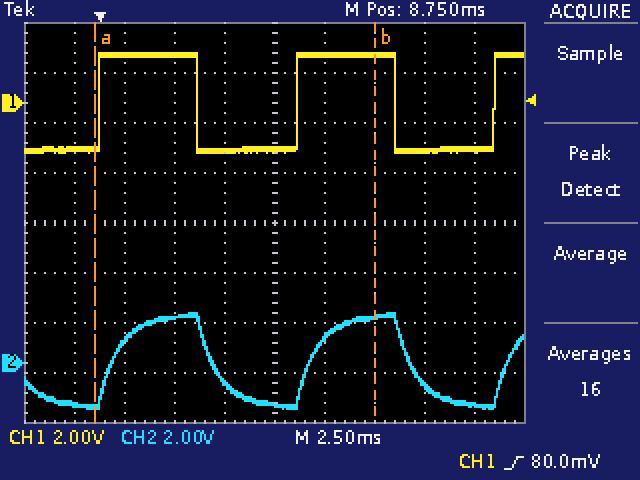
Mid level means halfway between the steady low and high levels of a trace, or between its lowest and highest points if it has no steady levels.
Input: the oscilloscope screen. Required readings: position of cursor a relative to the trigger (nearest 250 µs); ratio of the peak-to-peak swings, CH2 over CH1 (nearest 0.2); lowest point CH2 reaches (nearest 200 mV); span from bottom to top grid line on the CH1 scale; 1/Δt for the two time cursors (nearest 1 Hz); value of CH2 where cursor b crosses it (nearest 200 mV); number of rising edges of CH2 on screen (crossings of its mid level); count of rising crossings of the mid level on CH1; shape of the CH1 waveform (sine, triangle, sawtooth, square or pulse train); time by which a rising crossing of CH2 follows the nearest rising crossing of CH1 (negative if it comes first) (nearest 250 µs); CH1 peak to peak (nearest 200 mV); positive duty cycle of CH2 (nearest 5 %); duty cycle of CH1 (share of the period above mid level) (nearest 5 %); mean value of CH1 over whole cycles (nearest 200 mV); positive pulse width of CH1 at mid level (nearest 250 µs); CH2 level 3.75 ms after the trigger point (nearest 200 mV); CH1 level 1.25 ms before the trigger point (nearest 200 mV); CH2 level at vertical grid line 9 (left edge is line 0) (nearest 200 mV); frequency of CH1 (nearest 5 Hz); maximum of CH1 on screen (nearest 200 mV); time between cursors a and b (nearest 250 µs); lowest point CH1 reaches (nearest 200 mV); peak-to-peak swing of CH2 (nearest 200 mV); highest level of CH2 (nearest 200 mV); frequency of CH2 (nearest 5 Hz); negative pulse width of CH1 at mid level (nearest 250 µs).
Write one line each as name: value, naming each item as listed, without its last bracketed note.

position of cursor a relative to the trigger: -250 µs
ratio of the peak-to-peak swings, CH2 over CH1: 1.0
lowest point CH2 reaches: -1.8 V
span from bottom to top grid line on the CH1 scale: 16 V
1/Δt for the two time cursors: 71 Hz
value of CH2 where cursor b crosses it: 1.8 V
number of rising edges of CH2 on screen: 3
count of rising crossings of the mid level on CH1: 3
shape of the CH1 waveform: square
time by which a rising crossing of CH2 follows the nearest rising crossing of CH1 (negative if it comes first): +750 µs
CH1 peak to peak: 4.0 V
positive duty cycle of CH2: 50 %
duty cycle of CH1 (share of the period above mid level): 50 %
mean value of CH1 over whole cycles: 0.0 V
positive pulse width of CH1 at mid level: 5.00 ms
CH2 level 3.75 ms after the trigger point: 1.8 V
CH1 level 1.25 ms before the trigger point: -1.8 V
CH2 level at vertical grid line 9 (left edge is line 0): -1.6 V
frequency of CH1: 100 Hz
maximum of CH1 on screen: 2.0 V
time between cursors a and b: 14.00 ms
lowest point CH1 reaches: -2.0 V
peak-to-peak swing of CH2: 3.8 V
highest level of CH2: 2.0 V
frequency of CH2: 100 Hz
negative pulse width of CH1 at mid level: 5.00 ms
